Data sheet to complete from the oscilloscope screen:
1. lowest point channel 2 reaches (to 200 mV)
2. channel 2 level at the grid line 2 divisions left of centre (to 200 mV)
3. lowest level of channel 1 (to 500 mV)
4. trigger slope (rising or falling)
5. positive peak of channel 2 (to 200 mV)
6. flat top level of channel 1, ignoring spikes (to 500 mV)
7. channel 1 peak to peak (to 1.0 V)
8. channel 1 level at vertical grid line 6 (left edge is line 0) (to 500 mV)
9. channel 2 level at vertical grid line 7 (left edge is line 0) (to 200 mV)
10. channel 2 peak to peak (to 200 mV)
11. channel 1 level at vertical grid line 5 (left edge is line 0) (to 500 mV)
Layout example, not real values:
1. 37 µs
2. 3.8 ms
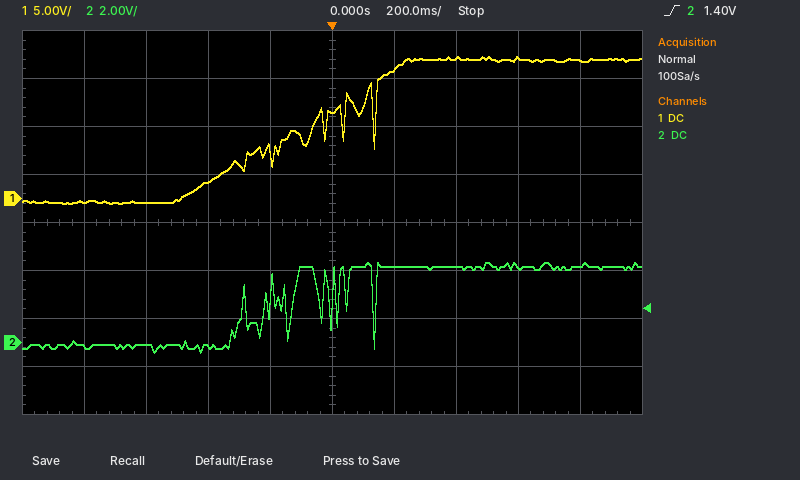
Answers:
1. -400 mV
2. -200 mV
3. -500 mV
4. rising
5. 3.4 V
6. 14.5 V
7. 15.0 V
8. 13.5 V
9. 3.2 V
10. 3.8 V
11. 9.0 V
